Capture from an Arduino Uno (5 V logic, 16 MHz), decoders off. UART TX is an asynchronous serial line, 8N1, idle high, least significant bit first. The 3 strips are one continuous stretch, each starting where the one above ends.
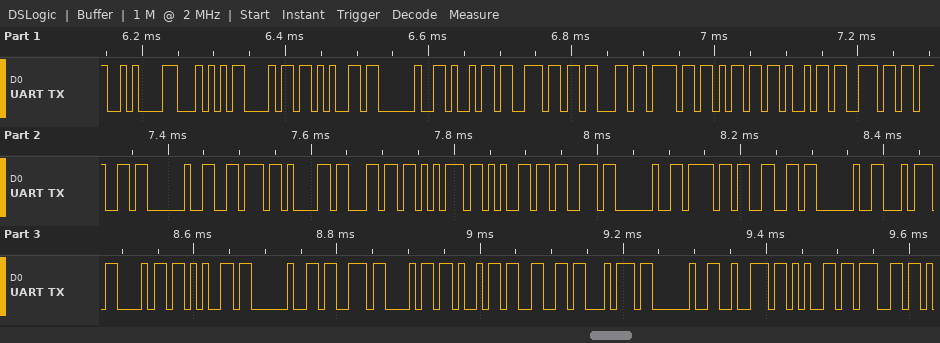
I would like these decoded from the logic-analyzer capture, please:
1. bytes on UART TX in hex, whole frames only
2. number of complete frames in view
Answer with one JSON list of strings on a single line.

["0A 54 68 65 20 69 6E 63 6F 6D 69 6E 67 20 76 61 6C 75 65 73 20 6F 66 20 74 68 65 20 73 68 69 66 74 20 72 65 67", "37"]
